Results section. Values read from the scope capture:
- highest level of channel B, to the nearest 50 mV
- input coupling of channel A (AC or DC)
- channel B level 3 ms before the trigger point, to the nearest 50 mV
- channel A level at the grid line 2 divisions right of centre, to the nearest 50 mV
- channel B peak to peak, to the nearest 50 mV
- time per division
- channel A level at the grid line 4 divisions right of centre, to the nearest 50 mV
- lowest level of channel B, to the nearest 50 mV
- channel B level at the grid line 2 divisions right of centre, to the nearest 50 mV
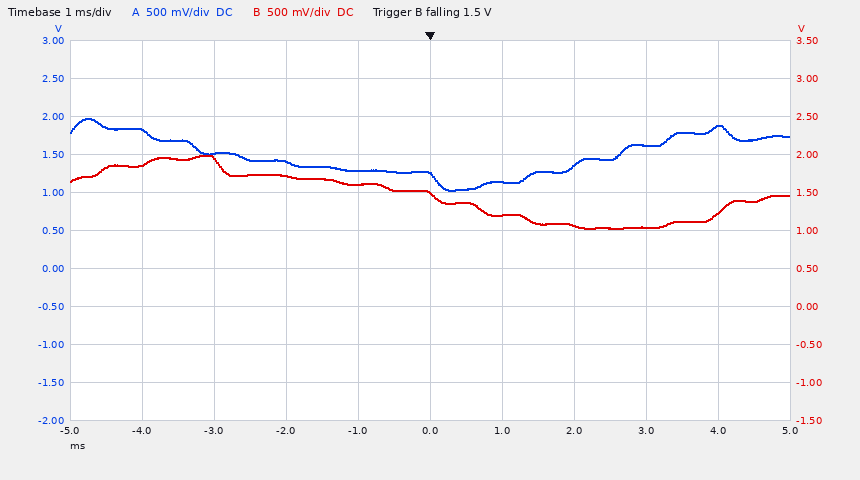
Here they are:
2.00 V
DC
1.95 V
1.35 V
950 mV
1 ms
1.85 V
1.05 V
1.05 V
